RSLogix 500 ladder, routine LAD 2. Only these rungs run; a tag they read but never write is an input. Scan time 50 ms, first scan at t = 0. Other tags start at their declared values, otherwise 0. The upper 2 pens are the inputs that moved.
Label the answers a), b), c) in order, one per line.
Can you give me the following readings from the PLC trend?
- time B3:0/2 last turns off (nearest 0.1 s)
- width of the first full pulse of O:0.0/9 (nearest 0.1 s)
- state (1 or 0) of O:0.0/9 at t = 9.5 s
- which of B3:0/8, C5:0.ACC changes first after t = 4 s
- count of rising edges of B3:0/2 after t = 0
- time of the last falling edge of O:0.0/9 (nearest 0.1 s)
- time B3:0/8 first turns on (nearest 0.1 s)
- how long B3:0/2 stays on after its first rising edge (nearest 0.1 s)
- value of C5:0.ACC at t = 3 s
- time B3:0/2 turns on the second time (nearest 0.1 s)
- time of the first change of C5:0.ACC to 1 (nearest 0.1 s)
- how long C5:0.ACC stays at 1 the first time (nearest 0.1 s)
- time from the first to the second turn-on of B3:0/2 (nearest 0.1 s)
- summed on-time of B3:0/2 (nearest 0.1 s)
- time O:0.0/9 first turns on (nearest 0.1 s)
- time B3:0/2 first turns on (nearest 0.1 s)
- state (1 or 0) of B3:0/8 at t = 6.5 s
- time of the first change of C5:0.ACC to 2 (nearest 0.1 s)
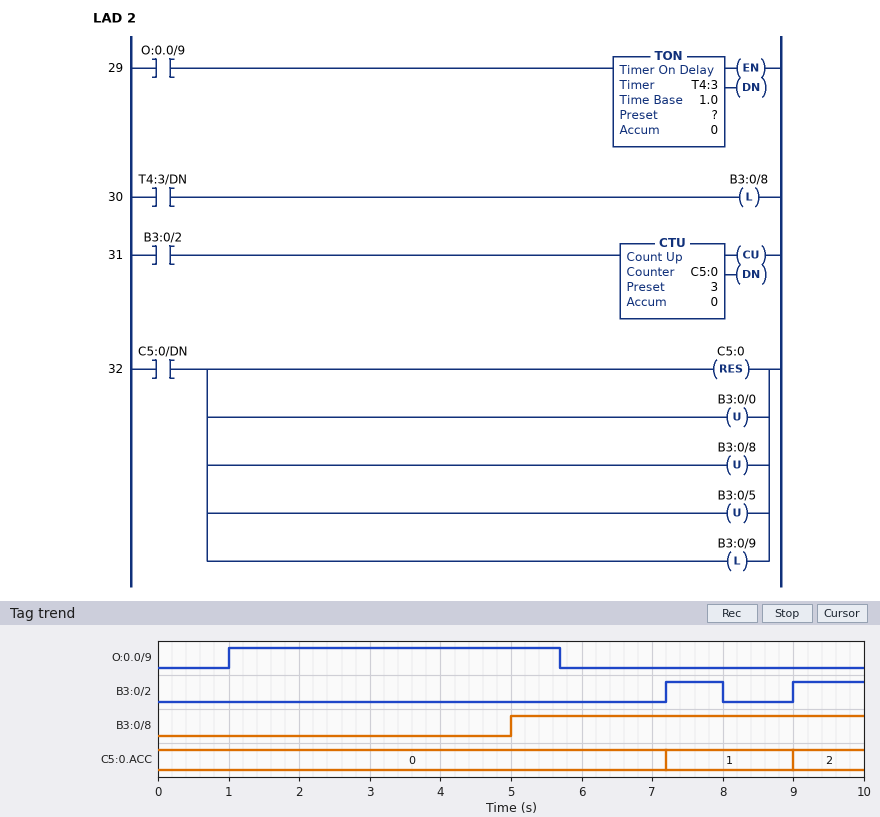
a) 8.0 s
b) 4.7 s
c) 0
d) B3:0/8
e) 2
f) 5.7 s
g) 5.0 s
h) 0.8 s
i) 0
j) 9.0 s
k) 7.2 s
l) 1.8 s
m) 1.8 s
n) 1.8 s
o) 1.0 s
p) 7.2 s
q) 1
r) 9.0 s
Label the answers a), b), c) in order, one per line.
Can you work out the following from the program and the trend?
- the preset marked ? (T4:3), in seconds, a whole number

a) 4 s
